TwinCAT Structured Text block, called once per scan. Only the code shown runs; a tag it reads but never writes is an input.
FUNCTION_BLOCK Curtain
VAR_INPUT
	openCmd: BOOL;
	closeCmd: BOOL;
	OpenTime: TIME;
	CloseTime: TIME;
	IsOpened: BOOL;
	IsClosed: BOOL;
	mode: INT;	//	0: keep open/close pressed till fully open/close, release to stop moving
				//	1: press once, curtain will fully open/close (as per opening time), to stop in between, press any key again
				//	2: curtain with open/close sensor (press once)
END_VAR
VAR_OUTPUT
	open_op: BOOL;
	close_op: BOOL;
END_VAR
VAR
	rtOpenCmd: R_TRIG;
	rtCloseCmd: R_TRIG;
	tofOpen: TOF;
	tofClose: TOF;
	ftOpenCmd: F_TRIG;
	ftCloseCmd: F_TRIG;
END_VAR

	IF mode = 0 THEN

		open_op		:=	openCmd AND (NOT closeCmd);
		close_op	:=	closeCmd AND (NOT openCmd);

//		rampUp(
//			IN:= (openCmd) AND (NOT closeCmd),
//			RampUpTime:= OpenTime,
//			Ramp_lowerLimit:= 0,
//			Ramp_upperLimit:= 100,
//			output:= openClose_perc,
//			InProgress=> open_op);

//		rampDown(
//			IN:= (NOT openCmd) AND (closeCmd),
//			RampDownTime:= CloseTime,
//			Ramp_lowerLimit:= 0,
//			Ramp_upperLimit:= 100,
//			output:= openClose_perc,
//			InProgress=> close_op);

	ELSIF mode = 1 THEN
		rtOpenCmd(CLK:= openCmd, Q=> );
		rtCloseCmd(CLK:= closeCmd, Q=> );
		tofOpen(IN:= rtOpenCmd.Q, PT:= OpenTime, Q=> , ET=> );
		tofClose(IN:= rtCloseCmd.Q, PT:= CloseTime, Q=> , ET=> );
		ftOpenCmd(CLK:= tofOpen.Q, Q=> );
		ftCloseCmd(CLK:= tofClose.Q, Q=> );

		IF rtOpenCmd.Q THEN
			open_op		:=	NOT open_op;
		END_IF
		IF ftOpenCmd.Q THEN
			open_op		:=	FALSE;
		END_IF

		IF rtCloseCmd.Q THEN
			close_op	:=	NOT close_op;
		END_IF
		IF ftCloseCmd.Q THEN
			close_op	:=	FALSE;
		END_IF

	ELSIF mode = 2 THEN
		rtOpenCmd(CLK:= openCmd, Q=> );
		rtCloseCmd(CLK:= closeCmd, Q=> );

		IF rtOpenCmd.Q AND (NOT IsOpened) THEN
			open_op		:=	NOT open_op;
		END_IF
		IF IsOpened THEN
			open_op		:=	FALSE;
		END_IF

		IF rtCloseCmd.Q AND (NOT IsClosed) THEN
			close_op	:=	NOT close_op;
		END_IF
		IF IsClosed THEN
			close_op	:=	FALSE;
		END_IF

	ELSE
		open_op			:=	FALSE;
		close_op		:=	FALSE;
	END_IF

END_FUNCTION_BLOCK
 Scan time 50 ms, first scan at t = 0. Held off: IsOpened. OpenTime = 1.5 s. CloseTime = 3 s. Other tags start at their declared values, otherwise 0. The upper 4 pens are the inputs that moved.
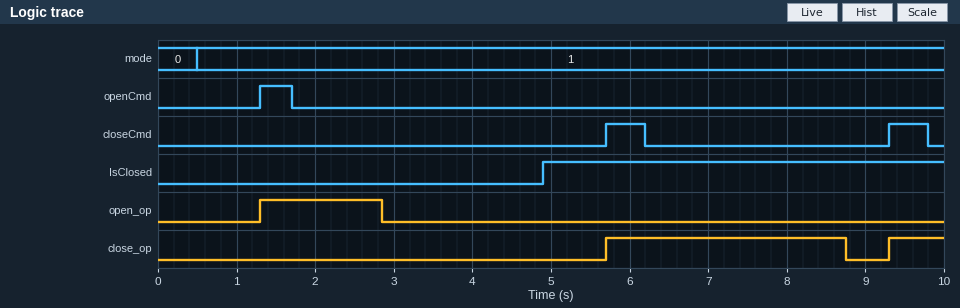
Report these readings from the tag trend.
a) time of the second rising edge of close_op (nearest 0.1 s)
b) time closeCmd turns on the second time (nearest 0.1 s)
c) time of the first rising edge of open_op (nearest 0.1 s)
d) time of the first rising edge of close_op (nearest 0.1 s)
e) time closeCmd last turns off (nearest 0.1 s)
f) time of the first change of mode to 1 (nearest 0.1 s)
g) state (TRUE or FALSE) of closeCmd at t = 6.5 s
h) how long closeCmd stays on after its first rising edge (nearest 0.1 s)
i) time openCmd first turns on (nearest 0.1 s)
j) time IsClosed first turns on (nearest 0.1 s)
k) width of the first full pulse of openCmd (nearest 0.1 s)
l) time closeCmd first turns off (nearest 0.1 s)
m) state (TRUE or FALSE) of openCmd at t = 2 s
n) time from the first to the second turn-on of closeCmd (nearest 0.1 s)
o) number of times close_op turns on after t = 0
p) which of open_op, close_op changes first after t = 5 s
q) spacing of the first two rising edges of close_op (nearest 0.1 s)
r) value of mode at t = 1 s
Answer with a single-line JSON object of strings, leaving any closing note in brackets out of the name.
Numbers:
{"time of the second rising edge of close_op": "9.3 s", "time closeCmd turns on the second time": "9.3 s", "time of the first rising edge of open_op": "1.3 s", "time of the first rising edge of close_op": "5.7 s", "time closeCmd last turns off": "9.8 s", "time of the first change of mode to 1": "0.5 s", "state (TRUE or FALSE) of closeCmd at t = 6.5 s": "FALSE", "how long closeCmd stays on after its first rising edge": "0.5 s", "time openCmd first turns on": "1.3 s", "time IsClosed first turns on": "4.9 s", "width of the first full pulse of openCmd": "0.4 s", "time closeCmd first turns off": "6.2 s", "state (TRUE or FALSE) of openCmd at t = 2 s": "FALSE", "time from the first to the second turn-on of closeCmd": "3.6 s", "number of times close_op turns on after t = 0": "2", "which of open_op, close_op changes first after t = 5 s": "close_op", "spacing of the first two rising edges of close_op": "3.6 s", "value of mode at t = 1 s": "1"}
